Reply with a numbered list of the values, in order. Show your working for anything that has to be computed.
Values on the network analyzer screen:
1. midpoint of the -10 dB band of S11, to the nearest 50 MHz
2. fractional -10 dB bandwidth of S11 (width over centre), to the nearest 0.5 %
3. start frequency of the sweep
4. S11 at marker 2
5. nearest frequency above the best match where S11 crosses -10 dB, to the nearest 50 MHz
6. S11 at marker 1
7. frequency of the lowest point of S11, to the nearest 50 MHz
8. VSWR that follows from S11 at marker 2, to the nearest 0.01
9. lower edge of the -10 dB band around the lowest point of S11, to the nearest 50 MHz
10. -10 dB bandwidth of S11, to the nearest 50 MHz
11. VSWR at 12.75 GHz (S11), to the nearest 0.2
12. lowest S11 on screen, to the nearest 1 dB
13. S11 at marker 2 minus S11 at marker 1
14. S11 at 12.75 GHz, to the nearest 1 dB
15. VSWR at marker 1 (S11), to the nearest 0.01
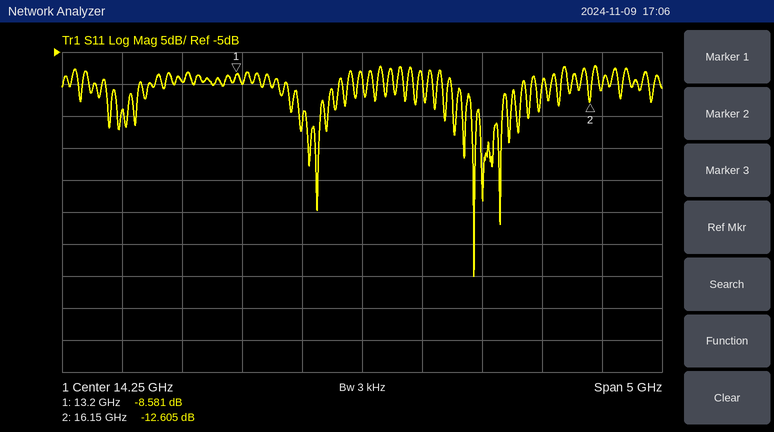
1. 15.30 GHz
2. 600 MHz / 15.3 GHz ≈ 3.92 %, so 4.0 % to the nearest 0.5 %
3. 11.75 GHz
4. -12.605 dB
5. 15.60 GHz
6. -8.581 dB
7. 15.20 GHz
8. (1 + 0.2343)/(1 − 0.2343) ≈ 1.61
9. 15.00 GHz
10. 15.60 GHz − 15.00 GHz = 600 MHz
11. |Γ| = 10^(-10/20) = 0.3162; VSWR = (1 + 0.3162)/(1 − 0.3162) ≈ 1.92, so 2.0 to the nearest 0.2
12. -40 dB
13. -12.605 − (-8.581) = -4.024 dB
14. -10 dB
15. (1 + 0.3723)/(1 − 0.3723) ≈ 2.19
